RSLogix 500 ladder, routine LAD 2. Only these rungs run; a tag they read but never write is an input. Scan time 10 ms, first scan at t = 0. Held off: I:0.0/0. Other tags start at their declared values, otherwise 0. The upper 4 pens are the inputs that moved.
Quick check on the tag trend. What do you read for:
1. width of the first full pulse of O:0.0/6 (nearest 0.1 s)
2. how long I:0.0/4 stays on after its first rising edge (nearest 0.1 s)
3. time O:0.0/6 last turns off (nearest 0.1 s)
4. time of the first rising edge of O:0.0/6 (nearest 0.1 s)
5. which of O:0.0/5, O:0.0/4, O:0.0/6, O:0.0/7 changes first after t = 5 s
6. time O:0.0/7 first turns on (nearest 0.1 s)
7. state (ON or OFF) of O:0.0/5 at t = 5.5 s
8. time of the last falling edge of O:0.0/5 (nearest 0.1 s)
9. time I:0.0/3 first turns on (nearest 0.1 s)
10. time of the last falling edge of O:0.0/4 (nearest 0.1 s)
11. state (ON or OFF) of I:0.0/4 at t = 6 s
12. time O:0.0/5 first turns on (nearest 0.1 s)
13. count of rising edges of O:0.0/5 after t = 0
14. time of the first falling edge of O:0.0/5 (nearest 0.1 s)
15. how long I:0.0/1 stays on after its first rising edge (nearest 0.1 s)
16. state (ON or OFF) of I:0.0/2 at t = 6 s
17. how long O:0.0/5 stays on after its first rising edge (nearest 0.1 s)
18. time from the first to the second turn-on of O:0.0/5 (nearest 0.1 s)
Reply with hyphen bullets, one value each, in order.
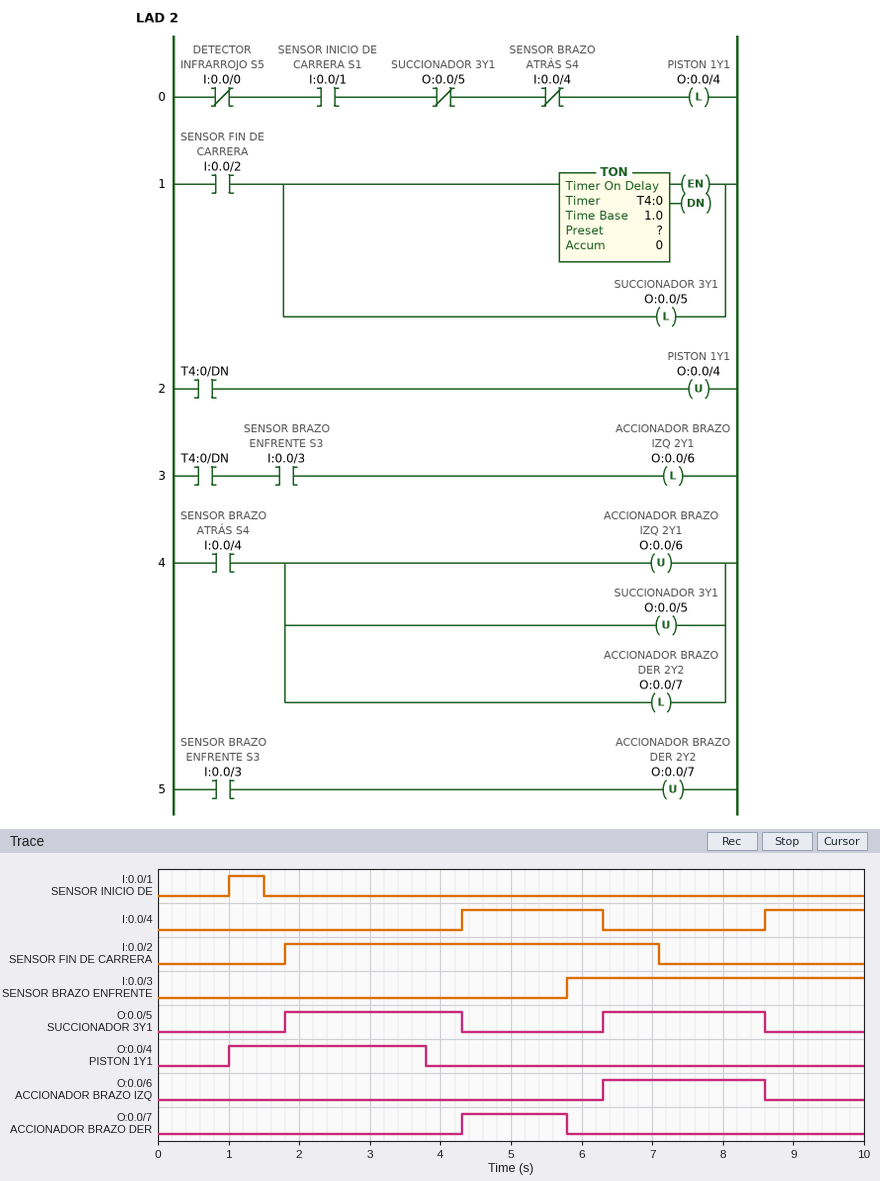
- 2.3 s
- 2.0 s
- 8.6 s
- 6.3 s
- O:0.0/7
- 4.3 s
- OFF
- 8.6 s
- 5.8 s
- 3.8 s
- ON
- 1.8 s
- 2
- 4.3 s
- 0.5 s
- ON
- 2.5 s
- 4.5 s
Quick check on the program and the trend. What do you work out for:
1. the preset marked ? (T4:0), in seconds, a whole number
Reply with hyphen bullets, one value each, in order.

- 2 s
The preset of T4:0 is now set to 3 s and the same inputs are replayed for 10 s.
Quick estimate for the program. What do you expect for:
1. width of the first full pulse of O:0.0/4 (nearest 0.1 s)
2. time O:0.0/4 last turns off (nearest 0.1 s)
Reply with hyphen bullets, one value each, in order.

- 3.8 s
- 4.8 s
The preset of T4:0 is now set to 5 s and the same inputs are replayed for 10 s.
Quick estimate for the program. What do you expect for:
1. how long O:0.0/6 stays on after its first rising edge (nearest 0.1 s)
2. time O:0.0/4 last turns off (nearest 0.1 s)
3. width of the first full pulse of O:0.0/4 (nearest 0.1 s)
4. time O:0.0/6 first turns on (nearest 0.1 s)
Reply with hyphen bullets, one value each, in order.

- 1.8 s
- 6.8 s
- 5.8 s
- 6.8 s
